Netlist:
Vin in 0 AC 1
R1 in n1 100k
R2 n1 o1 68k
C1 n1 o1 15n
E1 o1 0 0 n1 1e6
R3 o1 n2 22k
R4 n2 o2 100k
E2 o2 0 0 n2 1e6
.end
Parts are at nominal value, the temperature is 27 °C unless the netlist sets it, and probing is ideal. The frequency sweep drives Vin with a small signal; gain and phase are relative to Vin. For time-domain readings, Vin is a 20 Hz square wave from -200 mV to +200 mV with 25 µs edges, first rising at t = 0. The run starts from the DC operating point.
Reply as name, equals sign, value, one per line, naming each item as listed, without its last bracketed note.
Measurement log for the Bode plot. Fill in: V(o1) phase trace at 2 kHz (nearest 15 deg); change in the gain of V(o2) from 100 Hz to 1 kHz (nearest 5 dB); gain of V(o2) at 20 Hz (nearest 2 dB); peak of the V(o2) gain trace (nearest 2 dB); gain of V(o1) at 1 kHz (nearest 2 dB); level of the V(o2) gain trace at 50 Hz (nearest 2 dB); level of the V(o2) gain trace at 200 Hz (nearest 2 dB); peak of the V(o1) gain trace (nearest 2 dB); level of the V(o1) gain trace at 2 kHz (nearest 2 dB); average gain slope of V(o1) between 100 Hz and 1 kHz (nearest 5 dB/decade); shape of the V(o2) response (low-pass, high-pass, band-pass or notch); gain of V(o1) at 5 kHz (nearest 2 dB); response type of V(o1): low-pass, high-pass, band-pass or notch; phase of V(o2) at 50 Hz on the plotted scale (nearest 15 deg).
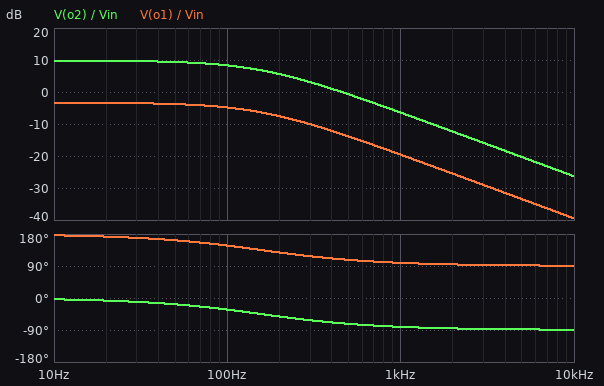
V(o1) phase trace at 2 kHz = 90 deg
change in the gain of V(o2) from 100 Hz to 1 kHz = -15 dB
gain of V(o2) at 20 Hz = 10 dB
peak of the V(o2) gain trace = 10 dB
gain of V(o1) at 1 kHz = -20 dB
level of the V(o2) gain trace at 50 Hz = 10 dB
level of the V(o2) gain trace at 200 Hz = 6 dB
peak of the V(o1) gain trace = -4 dB
level of the V(o1) gain trace at 2 kHz = -26 dB
average gain slope of V(o1) between 100 Hz and 1 kHz = -15 dB/decade
shape of the V(o2) response = low-pass
gain of V(o1) at 5 kHz = -34 dB
response type of V(o1): low-pass, high-pass, band-pass or notch = low-pass
phase of V(o2) at 50 Hz on the plotted scale = -15 deg
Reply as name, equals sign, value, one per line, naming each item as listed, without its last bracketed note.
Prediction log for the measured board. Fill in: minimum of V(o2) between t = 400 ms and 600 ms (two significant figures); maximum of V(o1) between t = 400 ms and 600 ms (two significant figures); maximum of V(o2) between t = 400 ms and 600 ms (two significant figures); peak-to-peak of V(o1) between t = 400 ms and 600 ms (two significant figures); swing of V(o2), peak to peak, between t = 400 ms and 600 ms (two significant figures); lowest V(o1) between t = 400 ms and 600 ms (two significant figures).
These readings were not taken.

minimum of V(o2) between t = 400 ms and 600 ms = -620 mV
maximum of V(o1) between t = 400 ms and 600 ms = 140 mV
maximum of V(o2) between t = 400 ms and 600 ms = 620 mV
peak-to-peak of V(o1) between t = 400 ms and 600 ms = 270 mV
swing of V(o2), peak to peak, between t = 400 ms and 600 ms = 1.2 V
lowest V(o1) between t = 400 ms and 600 ms = -140 mV
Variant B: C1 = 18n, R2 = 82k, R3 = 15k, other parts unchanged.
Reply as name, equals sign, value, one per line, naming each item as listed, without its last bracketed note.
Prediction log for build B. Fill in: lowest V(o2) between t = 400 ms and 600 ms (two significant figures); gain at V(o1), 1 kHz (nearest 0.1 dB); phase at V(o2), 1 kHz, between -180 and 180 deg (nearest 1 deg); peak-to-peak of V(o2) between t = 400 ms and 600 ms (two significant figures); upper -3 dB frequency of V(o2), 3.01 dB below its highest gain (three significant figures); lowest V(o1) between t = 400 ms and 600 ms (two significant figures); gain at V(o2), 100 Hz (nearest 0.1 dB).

lowest V(o2) between t = 400 ms and 600 ms = -1.1 V
gain at V(o1), 1 kHz = -21.1 dB
phase at V(o2), 1 kHz, between -180 and 180 deg = -84 deg
peak-to-peak of V(o2) between t = 400 ms and 600 ms = 2.2 V
upper -3 dB frequency of V(o2), 3.01 dB below its highest gain = 108 Hz
lowest V(o1) between t = 400 ms and 600 ms = -160 mV
gain at V(o2), 100 Hz = 12.1 dB
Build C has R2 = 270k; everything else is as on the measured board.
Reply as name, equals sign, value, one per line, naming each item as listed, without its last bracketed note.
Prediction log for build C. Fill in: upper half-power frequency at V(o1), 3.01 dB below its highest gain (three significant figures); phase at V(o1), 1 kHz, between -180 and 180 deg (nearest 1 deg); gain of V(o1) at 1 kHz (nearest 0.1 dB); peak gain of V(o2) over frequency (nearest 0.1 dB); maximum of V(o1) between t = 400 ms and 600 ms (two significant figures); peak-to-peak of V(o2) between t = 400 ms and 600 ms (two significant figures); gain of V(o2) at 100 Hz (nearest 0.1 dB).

upper half-power frequency at V(o1), 3.01 dB below its highest gain = 39.3 Hz
phase at V(o1), 1 kHz, between -180 and 180 deg = 92 deg
gain of V(o1) at 1 kHz = -19.5 dB
peak gain of V(o2) over frequency = 21.8 dB
maximum of V(o1) between t = 400 ms and 600 ms = 540 mV
peak-to-peak of V(o2) between t = 400 ms and 600 ms = 4.9 V
gain of V(o2) at 100 Hz = 13.0 dB
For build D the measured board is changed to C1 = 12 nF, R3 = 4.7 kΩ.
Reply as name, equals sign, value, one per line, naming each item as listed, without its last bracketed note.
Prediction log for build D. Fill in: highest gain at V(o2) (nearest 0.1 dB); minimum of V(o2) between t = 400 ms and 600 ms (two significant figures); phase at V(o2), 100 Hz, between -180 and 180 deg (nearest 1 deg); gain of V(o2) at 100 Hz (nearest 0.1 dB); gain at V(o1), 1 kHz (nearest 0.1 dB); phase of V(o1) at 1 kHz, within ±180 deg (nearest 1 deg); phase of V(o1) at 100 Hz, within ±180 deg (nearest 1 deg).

highest gain at V(o2) = 23.2 dB
minimum of V(o2) between t = 400 ms and 600 ms = -2.9 V
phase at V(o2), 100 Hz, between -180 and 180 deg = -27 deg
gain of V(o2) at 100 Hz = 22.2 dB
gain at V(o1), 1 kHz = -17.7 dB
phase of V(o1) at 1 kHz, within ±180 deg = 101 deg
phase of V(o1) at 100 Hz, within ±180 deg = 153 deg
